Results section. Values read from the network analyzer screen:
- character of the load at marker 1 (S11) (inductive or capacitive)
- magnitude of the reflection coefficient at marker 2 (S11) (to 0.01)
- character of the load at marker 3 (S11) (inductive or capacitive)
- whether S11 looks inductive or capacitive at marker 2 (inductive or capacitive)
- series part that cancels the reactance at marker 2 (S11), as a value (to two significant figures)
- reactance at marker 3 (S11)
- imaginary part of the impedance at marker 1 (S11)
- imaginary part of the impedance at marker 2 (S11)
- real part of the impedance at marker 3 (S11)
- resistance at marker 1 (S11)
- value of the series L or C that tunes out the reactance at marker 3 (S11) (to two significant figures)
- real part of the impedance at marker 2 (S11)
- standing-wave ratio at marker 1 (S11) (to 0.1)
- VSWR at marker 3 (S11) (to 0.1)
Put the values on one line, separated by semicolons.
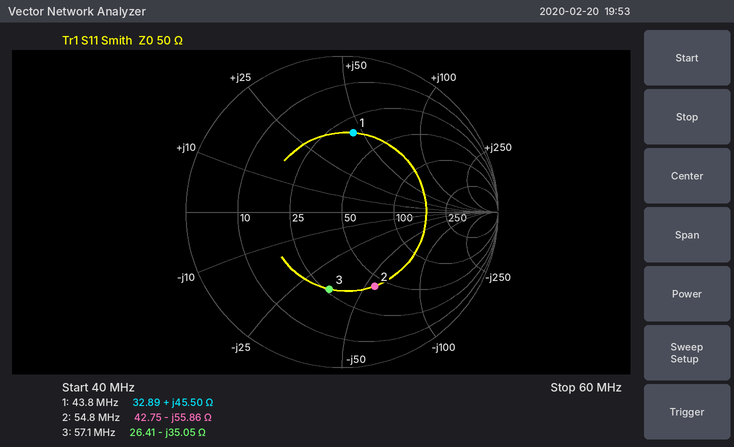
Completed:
inductive; 0.52; capacitive; capacitive; 160 nH; -35.05 Ω; +45.50 Ω; -55.86 Ω; 26.41 Ω; 32.89 Ω; 98 nH; 42.75 Ω; 3.1; 3.0
